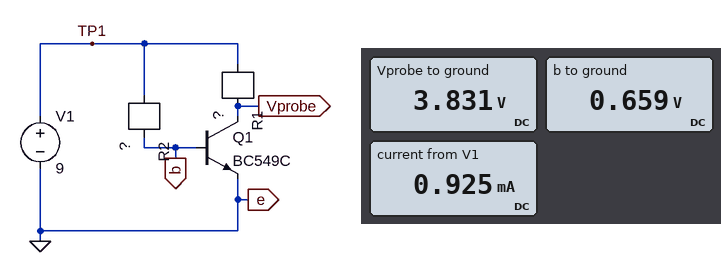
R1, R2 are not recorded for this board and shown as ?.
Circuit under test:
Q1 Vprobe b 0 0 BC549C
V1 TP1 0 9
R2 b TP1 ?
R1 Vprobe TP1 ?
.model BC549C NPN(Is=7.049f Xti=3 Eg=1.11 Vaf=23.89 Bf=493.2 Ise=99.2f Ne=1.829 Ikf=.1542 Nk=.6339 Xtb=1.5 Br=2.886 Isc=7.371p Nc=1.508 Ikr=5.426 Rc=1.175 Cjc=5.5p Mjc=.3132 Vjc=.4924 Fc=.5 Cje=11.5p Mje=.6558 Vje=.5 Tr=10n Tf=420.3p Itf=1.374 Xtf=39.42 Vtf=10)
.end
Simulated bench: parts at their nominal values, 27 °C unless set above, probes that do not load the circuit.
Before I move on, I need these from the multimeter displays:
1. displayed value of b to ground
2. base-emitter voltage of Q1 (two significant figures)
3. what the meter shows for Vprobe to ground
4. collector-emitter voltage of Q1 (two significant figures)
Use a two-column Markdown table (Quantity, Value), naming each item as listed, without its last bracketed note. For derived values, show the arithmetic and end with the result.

| Quantity | Value |
|---|---|
| displayed value of b to ground | 0.659 V |
| base-emitter voltage of Q1 | 659 mV = 660 mV |
| what the meter shows for Vprobe to ground | 3.831 V |
| collector-emitter voltage of Q1 | 3.831 V = 3.8 V |
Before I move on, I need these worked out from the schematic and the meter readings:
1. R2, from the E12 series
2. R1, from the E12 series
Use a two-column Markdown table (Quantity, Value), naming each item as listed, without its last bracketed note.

| Quantity | Value |
|---|---|
| R2, from the E12 series | 4.7 MΩ |
| R1, from the E12 series | 5.6 kΩ |
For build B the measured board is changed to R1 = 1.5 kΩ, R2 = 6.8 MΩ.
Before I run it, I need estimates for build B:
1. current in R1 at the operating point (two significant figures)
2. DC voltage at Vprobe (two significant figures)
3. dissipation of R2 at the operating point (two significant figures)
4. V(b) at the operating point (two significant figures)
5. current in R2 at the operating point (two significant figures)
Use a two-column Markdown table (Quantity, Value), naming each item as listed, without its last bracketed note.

| Quantity | Value |
|---|---|
| current in R1 at the operating point | 730 µA |
| DC voltage at Vprobe | 7.9 V |
| dissipation of R2 at the operating point | 10 µW |
| V(b) at the operating point | 650 mV |
| current in R2 at the operating point | 1.2 µA |
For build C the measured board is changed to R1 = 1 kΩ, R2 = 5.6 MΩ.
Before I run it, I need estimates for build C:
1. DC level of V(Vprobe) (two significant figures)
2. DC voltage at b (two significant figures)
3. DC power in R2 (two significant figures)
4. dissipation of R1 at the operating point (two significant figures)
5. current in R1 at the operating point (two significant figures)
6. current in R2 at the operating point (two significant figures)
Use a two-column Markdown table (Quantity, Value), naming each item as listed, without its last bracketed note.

| Quantity | Value |
|---|---|
| DC level of V(Vprobe) | 8.1 V |
| DC voltage at b | 650 mV |
| DC power in R2 | 12 µW |
| dissipation of R1 at the operating point | 800 µW |
| current in R1 at the operating point | 890 µA |
| current in R2 at the operating point | 1.5 µA |
